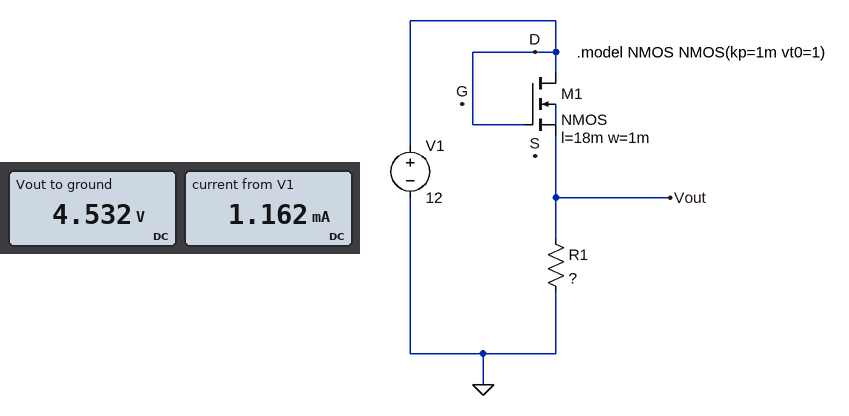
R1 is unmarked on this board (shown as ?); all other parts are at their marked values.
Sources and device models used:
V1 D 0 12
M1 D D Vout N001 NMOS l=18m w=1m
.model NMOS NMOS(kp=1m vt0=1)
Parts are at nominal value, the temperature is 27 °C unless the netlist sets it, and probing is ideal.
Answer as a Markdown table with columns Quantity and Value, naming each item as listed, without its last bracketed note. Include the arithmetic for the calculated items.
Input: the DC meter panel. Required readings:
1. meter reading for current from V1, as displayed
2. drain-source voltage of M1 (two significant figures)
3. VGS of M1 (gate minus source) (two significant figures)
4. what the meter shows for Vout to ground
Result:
| Quantity | Value |
|---|---|
| meter reading for current from V1, as displayed | 1.162 mA |
| drain-source voltage of M1 | 12 V - 4.532 V = 7.5 V |
| VGS of M1 (gate minus source) | 12 V - 4.532 V = 7.5 V |
| what the meter shows for Vout to ground | 4.532 V |
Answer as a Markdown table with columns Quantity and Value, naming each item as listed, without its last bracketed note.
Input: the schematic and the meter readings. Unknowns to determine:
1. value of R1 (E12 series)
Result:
| Quantity | Value |
|---|---|
| value of R1 | 3.9 kΩ |
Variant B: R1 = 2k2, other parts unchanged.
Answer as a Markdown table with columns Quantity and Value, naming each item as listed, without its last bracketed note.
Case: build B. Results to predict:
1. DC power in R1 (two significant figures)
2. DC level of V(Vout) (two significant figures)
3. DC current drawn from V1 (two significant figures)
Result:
| Quantity | Value |
|---|---|
| DC power in R1 | 5.5 mW |
| DC level of V(Vout) | 3.5 V |
| DC current drawn from V1 | 1.6 mA |
